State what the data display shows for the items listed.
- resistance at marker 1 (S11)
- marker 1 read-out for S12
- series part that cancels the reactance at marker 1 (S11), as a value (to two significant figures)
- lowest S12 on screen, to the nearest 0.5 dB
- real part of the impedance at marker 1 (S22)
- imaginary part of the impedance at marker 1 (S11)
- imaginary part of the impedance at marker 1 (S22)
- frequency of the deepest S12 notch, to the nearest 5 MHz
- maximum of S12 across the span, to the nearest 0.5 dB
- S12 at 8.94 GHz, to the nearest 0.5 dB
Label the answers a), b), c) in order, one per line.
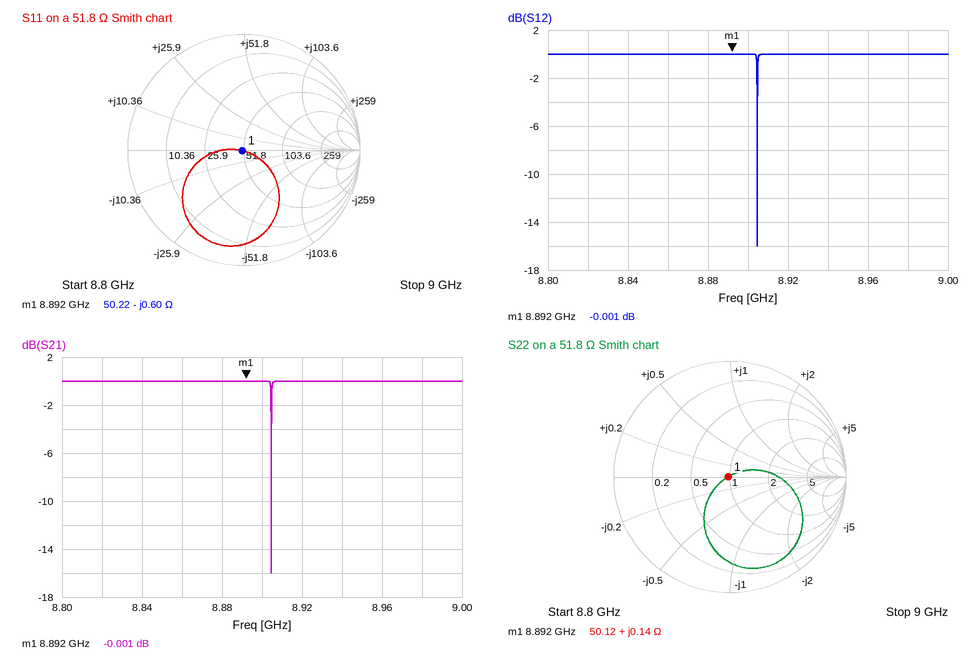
a) 50.22 Ω
b) -0.001 dB
c) 11 pH
d) -16.0 dB
e) 50.12 Ω
f) -0.60 Ω
g) +0.14 Ω
h) 8.905 GHz
i) 0.0 dB
j) 0.0 dB
